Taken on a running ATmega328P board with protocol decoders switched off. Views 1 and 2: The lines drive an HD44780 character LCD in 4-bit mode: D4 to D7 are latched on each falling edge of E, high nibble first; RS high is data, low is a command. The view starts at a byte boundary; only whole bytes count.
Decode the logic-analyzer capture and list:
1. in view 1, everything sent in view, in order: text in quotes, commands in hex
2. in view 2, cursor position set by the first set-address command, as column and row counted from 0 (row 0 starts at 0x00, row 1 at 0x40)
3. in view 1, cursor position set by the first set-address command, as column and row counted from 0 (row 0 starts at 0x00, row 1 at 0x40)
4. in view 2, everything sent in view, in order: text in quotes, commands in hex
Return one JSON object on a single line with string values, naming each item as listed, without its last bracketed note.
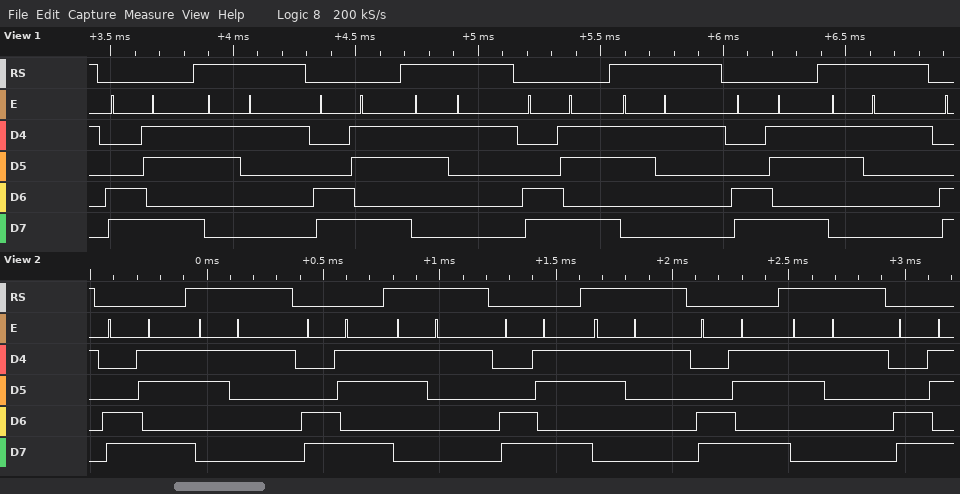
{"in view 1, everything sent in view, in order: text in quotes, commands in hex": "0xCB \"1\" 0xCB \"1\" 0xCB \"1\" 0xCB \"1\"", "in view 2, cursor position set by the first set-address command, as column and row counted from 0": "column 11, row 1", "in view 1, cursor position set by the first set-address command, as column and row counted from 0": "column 11, row 1", "in view 2, everything sent in view, in order: text in quotes, commands in hex": "0xCB \"1\" 0xCB \"1\" 0xCB \"1\" 0xCB \"1\" 0xCB"}
